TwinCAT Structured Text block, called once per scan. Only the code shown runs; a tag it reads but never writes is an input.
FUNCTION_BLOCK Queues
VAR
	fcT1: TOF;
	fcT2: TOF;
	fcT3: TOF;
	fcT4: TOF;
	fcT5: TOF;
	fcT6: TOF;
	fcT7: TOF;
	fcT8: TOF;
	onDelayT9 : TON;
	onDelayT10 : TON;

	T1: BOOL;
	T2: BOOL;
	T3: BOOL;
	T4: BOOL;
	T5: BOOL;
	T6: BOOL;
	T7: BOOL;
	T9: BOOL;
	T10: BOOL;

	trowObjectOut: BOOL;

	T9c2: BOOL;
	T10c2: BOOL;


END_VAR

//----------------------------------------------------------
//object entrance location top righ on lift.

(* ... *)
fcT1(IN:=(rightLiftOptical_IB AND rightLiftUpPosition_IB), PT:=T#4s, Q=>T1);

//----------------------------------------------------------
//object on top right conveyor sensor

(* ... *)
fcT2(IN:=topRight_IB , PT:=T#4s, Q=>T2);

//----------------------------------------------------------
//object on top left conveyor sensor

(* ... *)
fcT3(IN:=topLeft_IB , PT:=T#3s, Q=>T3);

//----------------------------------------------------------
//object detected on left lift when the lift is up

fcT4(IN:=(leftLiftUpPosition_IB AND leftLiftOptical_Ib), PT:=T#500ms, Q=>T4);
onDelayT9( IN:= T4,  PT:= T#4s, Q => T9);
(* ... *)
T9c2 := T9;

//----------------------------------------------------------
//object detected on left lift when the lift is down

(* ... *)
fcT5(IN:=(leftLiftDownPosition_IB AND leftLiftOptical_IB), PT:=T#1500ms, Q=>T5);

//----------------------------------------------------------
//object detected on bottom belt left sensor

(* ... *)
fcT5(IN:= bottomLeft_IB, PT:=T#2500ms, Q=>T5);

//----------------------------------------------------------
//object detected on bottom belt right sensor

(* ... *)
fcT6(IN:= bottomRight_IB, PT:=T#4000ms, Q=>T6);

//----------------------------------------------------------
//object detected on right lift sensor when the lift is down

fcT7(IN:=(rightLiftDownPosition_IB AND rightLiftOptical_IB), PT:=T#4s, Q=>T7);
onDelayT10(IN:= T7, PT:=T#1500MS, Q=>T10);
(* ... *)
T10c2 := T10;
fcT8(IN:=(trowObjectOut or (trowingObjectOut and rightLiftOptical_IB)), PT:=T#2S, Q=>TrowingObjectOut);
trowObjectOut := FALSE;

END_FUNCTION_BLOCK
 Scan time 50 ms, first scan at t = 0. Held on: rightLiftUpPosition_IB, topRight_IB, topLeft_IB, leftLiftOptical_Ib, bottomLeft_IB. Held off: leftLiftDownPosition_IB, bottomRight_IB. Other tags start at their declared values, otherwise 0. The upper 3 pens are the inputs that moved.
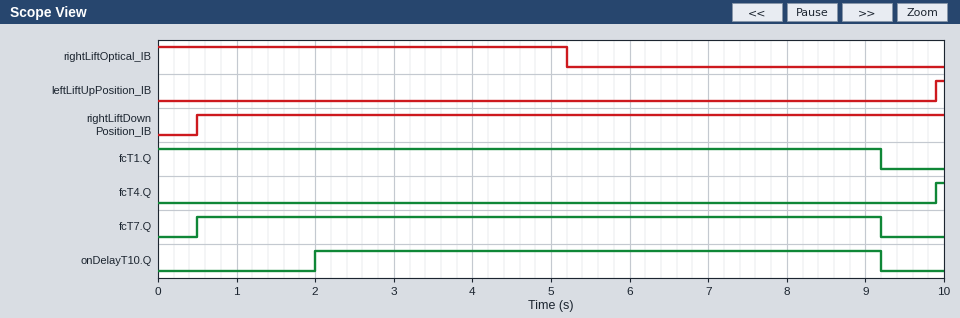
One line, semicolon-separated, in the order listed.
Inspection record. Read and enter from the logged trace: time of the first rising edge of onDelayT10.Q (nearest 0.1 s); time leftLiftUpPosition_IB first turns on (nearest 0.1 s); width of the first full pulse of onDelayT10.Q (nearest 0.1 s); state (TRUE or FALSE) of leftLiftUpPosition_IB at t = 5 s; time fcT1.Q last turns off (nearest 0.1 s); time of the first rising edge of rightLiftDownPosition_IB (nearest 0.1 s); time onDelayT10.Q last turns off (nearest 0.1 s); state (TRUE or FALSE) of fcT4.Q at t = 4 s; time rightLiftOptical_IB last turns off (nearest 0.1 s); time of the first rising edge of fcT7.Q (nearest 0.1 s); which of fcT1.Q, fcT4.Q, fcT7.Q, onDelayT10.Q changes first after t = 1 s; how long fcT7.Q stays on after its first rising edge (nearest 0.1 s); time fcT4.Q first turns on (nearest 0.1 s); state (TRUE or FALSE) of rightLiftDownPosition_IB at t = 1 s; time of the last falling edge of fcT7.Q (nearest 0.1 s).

2.0 s; 9.9 s; 7.2 s; FALSE; 9.2 s; 0.5 s; 9.2 s; FALSE; 5.2 s; 0.5 s; onDelayT10.Q; 8.7 s; 9.9 s; TRUE; 9.2 s
